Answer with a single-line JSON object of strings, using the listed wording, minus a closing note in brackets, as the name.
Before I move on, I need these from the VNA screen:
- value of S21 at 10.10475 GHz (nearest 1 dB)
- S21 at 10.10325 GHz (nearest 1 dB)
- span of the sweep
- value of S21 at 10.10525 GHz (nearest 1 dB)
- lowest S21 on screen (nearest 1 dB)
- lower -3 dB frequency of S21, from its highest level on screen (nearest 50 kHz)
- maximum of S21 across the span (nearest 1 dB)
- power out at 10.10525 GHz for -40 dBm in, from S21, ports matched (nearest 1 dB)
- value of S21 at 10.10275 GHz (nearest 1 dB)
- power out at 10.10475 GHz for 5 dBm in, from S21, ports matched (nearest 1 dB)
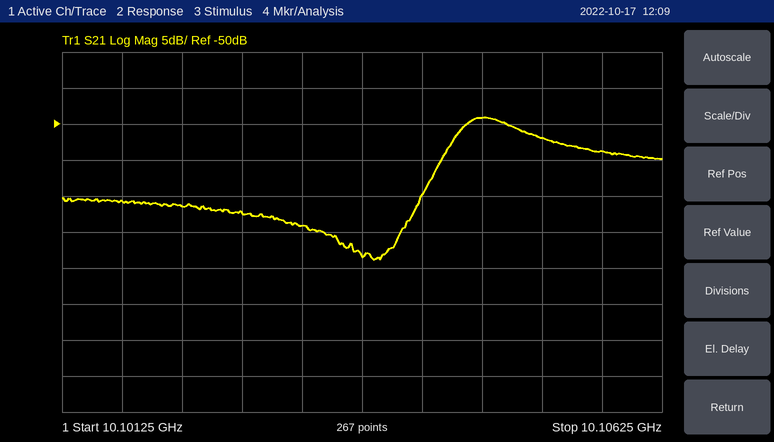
{"value of S21 at 10.10475 GHz": "-49 dB", "S21 at 10.10325 GHz": "-64 dB", "span of the sweep": "5 MHz", "value of S21 at 10.10525 GHz": "-52 dB", "lowest S21 on screen": "-69 dB", "lower -3 dB frequency of S21, from its highest level on screen": "10.10450 GHz", "maximum of S21 across the span": "-49 dB", "power out at 10.10525 GHz for -40 dBm in, from S21, ports matched": "-92 dBm", "value of S21 at 10.10275 GHz": "-62 dB", "power out at 10.10475 GHz for 5 dBm in, from S21, ports matched": "-44 dBm"}
